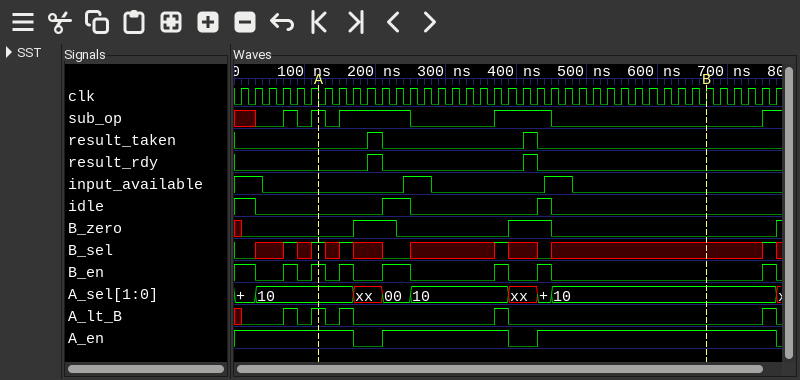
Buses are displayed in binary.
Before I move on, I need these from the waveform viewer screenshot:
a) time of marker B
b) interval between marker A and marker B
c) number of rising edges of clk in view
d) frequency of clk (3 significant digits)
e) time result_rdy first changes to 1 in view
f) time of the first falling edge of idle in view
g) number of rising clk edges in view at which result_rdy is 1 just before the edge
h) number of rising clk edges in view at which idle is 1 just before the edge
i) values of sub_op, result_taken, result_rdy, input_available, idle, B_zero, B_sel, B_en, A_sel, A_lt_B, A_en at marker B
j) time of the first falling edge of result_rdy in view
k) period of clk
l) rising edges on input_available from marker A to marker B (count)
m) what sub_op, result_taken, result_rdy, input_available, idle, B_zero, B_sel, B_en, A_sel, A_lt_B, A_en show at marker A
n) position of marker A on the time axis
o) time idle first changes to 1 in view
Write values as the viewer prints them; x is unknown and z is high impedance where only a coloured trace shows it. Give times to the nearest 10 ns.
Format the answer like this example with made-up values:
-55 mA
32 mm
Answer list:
670 ns
550 ns
39
50.0 MHz
190 ns
30 ns
2
5
sub_op=0, result_taken=0, result_rdy=0, input_available=0, idle=0, B_zero=0, B_sel=x, B_en=0, A_sel=10, A_lt_B=0, A_en=1
210 ns
20 ns
2
sub_op=1, result_taken=0, result_rdy=0, input_available=0, idle=0, B_zero=0, B_sel=1, B_en=1, A_sel=10, A_lt_B=1, A_en=1
120 ns
210 ns
